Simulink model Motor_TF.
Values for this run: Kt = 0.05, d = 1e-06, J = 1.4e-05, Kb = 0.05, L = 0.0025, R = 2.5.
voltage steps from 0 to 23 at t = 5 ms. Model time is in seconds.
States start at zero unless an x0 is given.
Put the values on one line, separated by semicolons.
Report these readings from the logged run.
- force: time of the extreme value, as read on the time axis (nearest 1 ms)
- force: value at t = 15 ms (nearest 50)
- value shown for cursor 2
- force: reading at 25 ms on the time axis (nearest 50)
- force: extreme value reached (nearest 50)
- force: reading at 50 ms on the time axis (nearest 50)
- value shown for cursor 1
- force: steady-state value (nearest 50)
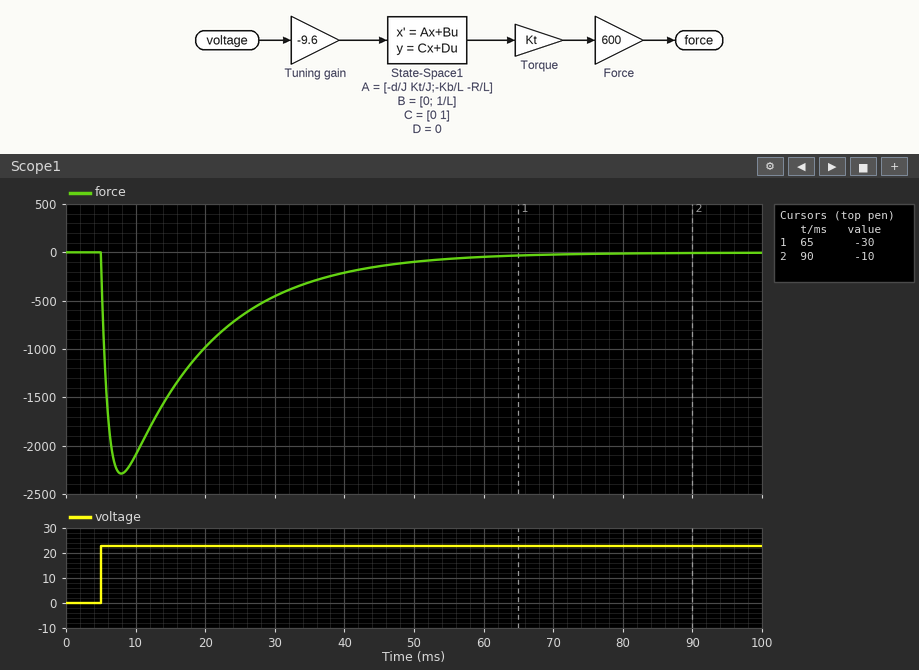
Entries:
8 ms; -1450; -10; -650; -2300; -100; -30; 0
